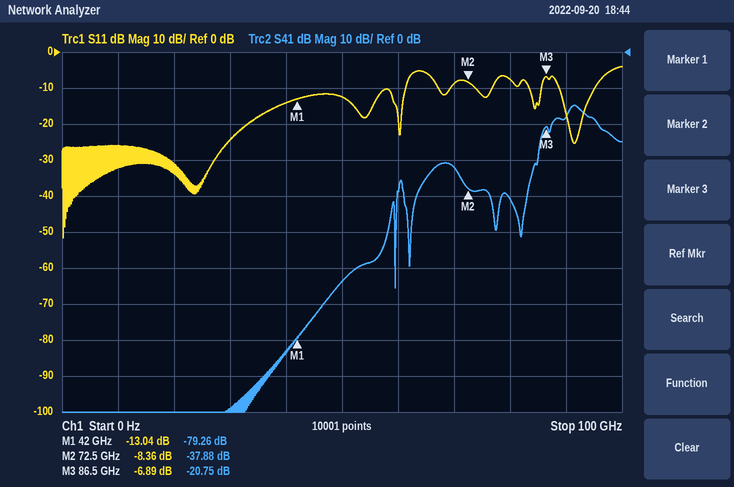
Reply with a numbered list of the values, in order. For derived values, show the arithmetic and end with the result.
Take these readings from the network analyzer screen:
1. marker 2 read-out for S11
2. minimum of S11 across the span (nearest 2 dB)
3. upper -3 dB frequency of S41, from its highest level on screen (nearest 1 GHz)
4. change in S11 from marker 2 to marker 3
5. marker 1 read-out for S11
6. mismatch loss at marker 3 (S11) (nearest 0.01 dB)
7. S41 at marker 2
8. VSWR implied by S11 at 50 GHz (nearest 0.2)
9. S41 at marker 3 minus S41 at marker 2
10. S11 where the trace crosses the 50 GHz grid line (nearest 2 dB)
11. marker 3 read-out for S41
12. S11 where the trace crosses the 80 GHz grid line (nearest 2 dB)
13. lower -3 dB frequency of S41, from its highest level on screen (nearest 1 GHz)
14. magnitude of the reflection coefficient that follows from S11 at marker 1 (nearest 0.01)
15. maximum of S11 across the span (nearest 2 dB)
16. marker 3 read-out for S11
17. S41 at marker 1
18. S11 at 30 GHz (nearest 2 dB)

1. -8.36 dB
2. -52 dB
3. 94 GHz
4. -6.89 − (-8.36) = 1.47 dB
5. -13.04 dB
6. −10 log10(1 − 10^(-6.89/10)) ≈ 0.99 dB
7. -37.88 dB
8. |Γ| = 10^(-12/20) = 0.2512; VSWR = (1 + 0.2512)/(1 − 0.2512) ≈ 1.67, so 1.6 to the nearest 0.2
9. -20.75 − (-37.88) = 17.13 dB
10. -12 dB
11. -20.75 dB
12. -8 dB
13. 90 GHz
14. 10^(-13.04/20) ≈ 0.22
15. -4 dB
16. -6.89 dB
17. -79.26 dB
18. -24 dB
